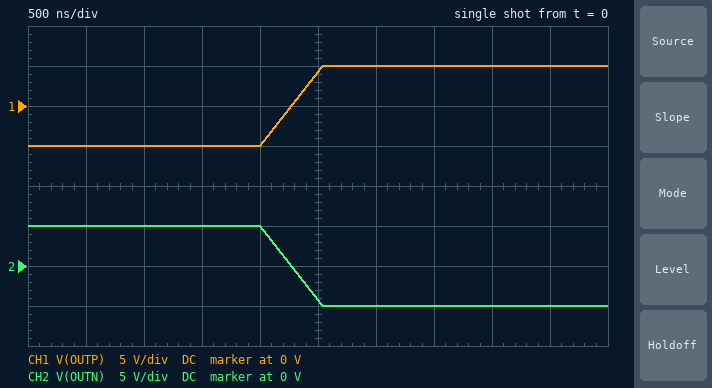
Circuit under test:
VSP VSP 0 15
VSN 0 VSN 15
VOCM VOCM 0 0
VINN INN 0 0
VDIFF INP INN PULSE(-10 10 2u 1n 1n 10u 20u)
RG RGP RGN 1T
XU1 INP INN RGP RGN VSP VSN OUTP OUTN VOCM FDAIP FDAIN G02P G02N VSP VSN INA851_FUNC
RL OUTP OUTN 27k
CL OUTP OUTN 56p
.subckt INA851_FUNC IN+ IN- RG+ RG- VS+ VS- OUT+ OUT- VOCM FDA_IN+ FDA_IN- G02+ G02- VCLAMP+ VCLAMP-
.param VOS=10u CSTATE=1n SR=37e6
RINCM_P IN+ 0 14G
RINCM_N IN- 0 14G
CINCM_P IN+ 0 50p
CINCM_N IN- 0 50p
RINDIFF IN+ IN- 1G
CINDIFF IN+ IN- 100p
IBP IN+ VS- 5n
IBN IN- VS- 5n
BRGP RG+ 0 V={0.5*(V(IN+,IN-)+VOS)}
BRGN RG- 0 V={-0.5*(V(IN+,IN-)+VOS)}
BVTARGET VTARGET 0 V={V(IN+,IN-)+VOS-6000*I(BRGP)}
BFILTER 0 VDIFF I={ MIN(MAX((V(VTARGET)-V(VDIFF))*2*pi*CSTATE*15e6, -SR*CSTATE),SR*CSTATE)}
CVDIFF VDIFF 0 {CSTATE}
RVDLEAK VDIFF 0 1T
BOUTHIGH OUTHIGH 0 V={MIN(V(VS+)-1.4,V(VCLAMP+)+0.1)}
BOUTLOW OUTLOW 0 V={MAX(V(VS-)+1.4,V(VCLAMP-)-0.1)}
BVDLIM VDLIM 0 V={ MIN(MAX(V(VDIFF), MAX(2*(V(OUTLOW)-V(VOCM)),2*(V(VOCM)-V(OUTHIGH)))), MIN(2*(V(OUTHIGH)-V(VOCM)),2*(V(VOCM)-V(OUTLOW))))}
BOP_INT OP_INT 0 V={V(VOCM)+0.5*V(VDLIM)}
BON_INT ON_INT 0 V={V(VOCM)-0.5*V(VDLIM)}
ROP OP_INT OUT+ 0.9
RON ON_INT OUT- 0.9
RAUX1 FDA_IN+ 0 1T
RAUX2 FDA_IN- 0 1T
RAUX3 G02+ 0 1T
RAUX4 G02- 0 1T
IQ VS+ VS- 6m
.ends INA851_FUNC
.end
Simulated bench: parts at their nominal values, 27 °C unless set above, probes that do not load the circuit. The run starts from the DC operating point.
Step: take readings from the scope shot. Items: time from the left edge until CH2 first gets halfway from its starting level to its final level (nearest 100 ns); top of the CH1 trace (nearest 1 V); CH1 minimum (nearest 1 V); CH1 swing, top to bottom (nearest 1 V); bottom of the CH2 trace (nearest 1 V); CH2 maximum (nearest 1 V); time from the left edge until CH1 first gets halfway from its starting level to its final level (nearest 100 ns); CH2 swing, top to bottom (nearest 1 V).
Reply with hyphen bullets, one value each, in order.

- 2.3 µs
- 5 V
- -5 V
- 10 V
- -5 V
- 5 V
- 2.3 µs
- 10 V
